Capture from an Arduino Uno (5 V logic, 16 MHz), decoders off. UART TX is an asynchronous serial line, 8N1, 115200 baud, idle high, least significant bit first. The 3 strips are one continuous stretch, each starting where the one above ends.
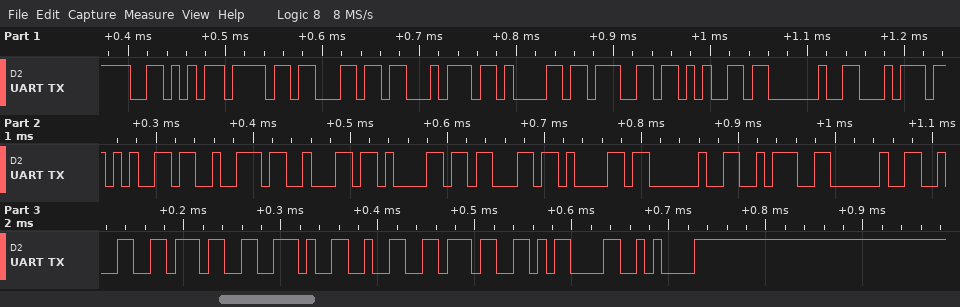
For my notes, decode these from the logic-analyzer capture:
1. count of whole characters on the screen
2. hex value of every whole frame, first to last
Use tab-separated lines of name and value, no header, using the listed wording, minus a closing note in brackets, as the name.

count of whole characters on the screen	25
hex value of every whole frame, first to last	56 6F 6C 74 61 67 65 20 74 65 72 62 61 63 61 20 3A 20 32 37 2E 32 37 0D 0A
